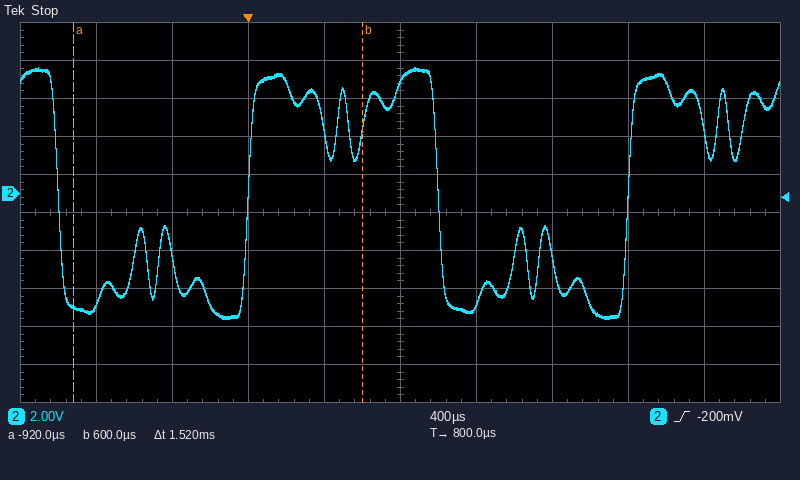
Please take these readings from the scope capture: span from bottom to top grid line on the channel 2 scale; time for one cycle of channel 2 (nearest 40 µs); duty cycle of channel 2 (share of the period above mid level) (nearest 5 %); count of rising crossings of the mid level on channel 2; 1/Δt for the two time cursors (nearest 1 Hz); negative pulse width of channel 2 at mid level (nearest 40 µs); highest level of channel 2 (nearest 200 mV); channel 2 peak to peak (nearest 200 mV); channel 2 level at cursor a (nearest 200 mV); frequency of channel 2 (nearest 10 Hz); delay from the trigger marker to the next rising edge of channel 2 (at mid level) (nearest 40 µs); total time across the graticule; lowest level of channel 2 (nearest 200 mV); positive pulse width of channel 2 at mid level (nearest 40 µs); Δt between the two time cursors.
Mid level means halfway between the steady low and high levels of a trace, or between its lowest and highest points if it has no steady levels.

20 V
2.00 ms
50 %
2
658 Hz
1.00 ms
6.6 V
13.2 V
-6.0 V
500 Hz
2.00 ms
4 ms
-6.6 V
1.00 ms
1.52 ms
